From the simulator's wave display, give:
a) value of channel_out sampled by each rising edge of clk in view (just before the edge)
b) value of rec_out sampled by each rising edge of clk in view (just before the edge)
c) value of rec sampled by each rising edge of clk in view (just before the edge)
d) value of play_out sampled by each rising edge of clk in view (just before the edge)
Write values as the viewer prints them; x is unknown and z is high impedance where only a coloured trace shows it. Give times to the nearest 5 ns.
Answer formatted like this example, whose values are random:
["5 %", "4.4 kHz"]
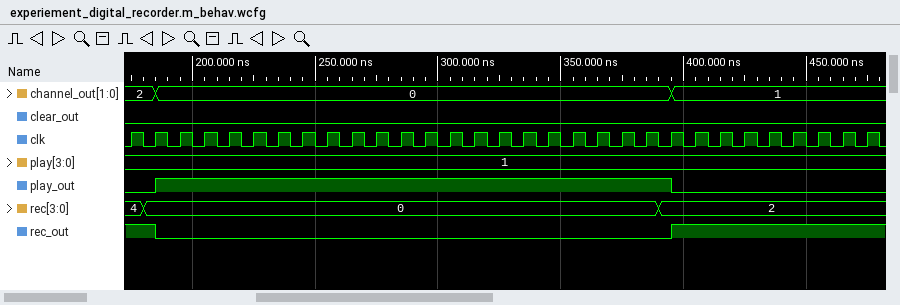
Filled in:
["2, 2, 0, 0, 0, 0, 0, 0, 0, 0, 0, 0, 0, 0, 0, 0, 0, 0, 0, 0, 0, 0, 0, 1, 1, 1, 1, 1, 1, 1, 1", "1 1 0 0 0 0 0 0 0 0 0 0 0 0 0 0 0 0 0 0 0 0 0 1 1 1 1 1 1 1 1", "4, 0, 0, 0, 0, 0, 0, 0, 0, 0, 0, 0, 0, 0, 0, 0, 0, 0, 0, 0, 0, 0, 2, 2, 2, 2, 2, 2, 2, 2, 2", "0 0 1 1 1 1 1 1 1 1 1 1 1 1 1 1 1 1 1 1 1 1 1 0 0 0 0 0 0 0 0"]
